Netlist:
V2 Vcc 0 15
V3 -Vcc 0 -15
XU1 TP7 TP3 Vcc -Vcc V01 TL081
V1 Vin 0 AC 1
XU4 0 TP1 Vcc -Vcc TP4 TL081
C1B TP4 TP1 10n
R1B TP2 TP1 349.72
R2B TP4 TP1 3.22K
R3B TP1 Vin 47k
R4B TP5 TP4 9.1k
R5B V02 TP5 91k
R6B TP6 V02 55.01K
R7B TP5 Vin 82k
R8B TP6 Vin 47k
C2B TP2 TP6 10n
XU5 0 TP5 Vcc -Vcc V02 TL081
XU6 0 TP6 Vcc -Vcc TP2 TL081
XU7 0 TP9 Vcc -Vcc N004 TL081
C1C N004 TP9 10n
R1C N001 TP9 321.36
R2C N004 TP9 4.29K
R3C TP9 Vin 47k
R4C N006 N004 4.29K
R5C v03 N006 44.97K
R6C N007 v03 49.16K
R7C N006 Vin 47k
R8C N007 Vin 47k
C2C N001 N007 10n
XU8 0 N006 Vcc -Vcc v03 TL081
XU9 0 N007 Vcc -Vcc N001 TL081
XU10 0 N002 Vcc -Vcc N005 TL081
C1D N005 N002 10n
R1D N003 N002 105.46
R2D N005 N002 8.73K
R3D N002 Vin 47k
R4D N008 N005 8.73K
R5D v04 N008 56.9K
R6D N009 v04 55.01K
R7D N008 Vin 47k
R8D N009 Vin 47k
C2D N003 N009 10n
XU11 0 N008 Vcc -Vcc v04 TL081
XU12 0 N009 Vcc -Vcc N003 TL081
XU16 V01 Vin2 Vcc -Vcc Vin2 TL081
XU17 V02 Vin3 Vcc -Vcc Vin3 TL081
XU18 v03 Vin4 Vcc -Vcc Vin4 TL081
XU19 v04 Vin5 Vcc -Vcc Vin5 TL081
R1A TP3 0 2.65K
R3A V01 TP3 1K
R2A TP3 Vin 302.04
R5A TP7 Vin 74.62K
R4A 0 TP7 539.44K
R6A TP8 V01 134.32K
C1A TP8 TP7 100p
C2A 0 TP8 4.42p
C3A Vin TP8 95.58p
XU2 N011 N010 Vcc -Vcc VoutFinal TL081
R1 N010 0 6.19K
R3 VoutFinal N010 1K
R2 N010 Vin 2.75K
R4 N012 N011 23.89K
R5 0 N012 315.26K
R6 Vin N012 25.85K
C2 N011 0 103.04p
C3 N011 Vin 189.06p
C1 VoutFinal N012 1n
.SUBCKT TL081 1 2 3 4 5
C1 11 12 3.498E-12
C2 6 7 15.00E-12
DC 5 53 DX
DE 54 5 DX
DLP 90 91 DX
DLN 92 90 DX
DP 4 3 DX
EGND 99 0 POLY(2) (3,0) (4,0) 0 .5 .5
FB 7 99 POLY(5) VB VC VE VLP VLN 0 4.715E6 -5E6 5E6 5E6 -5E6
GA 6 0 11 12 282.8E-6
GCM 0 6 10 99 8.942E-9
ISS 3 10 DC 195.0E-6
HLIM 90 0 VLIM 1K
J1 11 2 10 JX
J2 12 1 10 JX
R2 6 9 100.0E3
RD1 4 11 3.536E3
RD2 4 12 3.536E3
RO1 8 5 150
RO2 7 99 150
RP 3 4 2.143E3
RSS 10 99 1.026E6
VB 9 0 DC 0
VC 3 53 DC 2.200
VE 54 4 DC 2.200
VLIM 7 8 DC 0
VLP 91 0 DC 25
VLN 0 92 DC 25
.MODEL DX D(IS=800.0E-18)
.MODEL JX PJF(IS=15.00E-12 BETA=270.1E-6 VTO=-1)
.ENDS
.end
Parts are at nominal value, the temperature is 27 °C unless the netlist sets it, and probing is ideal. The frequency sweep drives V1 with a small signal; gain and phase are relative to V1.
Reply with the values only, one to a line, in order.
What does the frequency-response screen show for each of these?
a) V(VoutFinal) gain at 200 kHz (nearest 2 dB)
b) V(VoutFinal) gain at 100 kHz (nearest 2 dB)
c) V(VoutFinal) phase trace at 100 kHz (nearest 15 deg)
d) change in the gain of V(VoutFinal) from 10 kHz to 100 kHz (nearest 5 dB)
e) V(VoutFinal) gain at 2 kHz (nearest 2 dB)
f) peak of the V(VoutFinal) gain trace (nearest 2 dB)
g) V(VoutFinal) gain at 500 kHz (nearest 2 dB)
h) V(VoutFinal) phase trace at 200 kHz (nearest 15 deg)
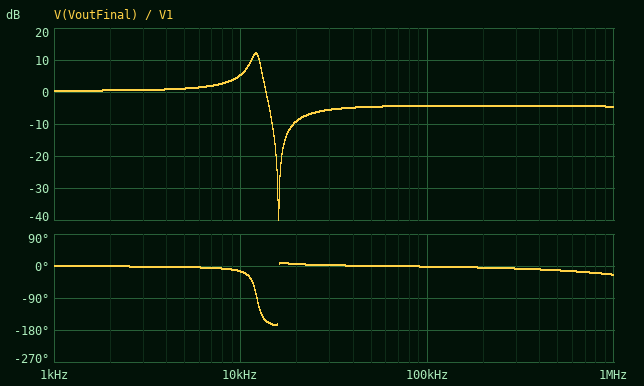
-4 dB
-4 dB
0 deg
-10 dB
0 dB
12 dB
-4 dB
0 deg
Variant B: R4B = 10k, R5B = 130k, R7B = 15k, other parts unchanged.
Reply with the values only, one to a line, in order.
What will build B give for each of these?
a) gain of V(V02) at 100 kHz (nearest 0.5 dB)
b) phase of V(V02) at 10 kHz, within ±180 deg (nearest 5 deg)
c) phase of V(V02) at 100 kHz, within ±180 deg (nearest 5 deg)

17.5 dB
-60 deg
145 deg
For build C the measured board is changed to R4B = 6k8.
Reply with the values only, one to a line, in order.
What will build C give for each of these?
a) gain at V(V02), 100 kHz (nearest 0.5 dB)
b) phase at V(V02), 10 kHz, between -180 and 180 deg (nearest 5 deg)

0 dB
155 deg
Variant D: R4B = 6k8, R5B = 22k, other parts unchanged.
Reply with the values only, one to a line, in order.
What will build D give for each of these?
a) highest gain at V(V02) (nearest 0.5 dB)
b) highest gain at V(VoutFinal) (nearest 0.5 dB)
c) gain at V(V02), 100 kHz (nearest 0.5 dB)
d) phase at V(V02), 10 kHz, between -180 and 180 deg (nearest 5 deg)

3.0 dB
12.0 dB
-11.5 dB
45 deg
